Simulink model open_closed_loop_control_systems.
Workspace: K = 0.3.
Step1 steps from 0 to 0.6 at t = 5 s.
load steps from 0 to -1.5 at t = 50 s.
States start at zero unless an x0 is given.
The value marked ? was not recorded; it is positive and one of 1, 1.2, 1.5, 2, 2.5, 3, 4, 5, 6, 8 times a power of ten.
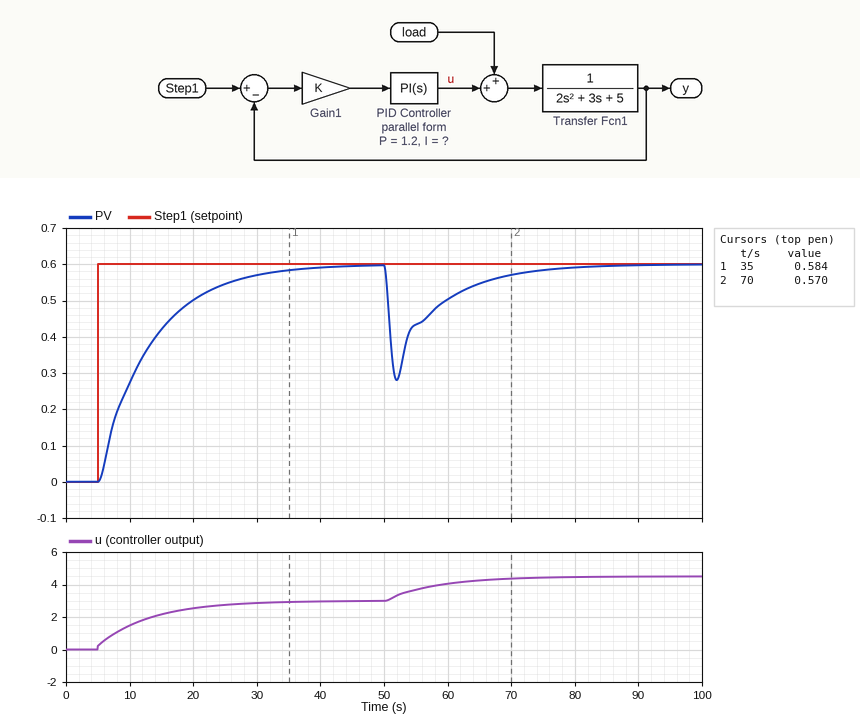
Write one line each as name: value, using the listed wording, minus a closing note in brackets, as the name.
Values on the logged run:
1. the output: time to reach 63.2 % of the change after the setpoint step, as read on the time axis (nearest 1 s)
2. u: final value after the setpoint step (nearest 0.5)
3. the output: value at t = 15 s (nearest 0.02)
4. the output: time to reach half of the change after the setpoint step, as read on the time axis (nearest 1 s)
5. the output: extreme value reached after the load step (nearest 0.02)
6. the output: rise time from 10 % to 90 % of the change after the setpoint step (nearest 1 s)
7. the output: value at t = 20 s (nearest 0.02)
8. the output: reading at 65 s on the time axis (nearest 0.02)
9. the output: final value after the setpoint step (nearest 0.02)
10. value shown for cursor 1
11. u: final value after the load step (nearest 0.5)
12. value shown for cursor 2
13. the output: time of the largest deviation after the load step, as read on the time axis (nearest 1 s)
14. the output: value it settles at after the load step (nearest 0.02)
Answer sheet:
the output: time to reach 63.2 % of the change after the setpoint step, as read on the time axis: 13 s
u: final value after the setpoint step: 3.0
the output: value at t = 15 s: 0.42
the output: time to reach half of the change after the setpoint step, as read on the time axis: 11 s
the output: extreme value reached after the load step: 0.28
the output: rise time from 10 % to 90 % of the change after the setpoint step: 18 s
the output: value at t = 20 s: 0.50
the output: reading at 65 s on the time axis: 0.54
the output: final value after the setpoint step: 0.60
value shown for cursor 1: 0.584
u: final value after the load step: 4.5
value shown for cursor 2: 0.570
the output: time of the largest deviation after the load step, as read on the time axis: 52 s
the output: value it settles at after the load step: 0.60
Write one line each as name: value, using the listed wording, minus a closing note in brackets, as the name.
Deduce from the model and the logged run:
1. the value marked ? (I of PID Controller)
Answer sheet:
the value marked ?: 2
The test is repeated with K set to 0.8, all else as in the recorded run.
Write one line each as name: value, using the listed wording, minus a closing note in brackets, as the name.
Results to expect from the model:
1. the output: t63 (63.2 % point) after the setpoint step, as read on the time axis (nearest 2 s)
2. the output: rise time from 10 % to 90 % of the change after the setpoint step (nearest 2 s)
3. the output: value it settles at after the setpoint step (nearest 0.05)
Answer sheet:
the output: t63 (63.2 % point) after the setpoint step, as read on the time axis: 8 s
the output: rise time from 10 % to 90 % of the change after the setpoint step: 6 s
the output: value it settles at after the setpoint step: 0.60
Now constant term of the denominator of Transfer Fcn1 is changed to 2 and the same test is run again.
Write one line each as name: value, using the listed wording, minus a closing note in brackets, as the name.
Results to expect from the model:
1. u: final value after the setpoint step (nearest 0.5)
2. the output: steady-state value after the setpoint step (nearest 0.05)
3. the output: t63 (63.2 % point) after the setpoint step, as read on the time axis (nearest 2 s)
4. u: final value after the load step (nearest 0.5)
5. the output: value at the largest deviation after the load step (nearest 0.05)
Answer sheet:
u: final value after the setpoint step: 1.0
the output: steady-state value after the setpoint step: 0.60
the output: t63 (63.2 % point) after the setpoint step, as read on the time axis: 8 s
u: final value after the load step: 2.5
the output: value at the largest deviation after the load step: 0.05
